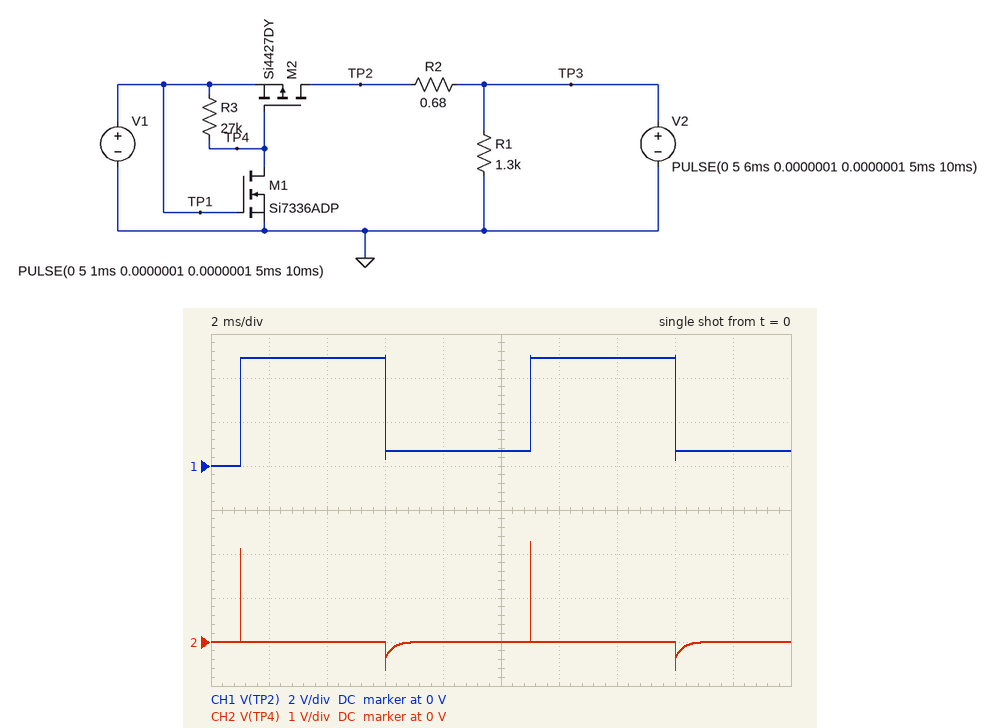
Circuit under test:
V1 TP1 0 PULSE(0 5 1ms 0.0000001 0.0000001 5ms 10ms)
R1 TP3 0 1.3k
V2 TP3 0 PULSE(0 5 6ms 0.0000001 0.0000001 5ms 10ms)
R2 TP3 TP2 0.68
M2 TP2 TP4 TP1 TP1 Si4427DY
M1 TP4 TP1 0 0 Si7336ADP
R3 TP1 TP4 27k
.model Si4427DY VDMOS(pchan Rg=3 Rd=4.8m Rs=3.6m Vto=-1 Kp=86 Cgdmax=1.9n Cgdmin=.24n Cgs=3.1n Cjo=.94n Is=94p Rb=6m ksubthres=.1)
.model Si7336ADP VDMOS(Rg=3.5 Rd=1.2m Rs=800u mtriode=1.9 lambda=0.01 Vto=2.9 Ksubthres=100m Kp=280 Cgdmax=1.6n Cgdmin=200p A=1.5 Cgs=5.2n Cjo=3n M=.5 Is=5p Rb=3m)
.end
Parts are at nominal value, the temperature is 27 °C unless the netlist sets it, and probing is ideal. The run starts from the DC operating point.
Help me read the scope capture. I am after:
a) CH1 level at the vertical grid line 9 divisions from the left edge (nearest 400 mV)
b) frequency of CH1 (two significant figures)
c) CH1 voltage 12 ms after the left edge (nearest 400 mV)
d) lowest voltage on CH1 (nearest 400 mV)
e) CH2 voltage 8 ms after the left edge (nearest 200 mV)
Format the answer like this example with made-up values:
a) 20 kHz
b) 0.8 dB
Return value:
a) 800 mV
b) 100 Hz
c) 4.8 V
d) 0 V
e) 0 V
